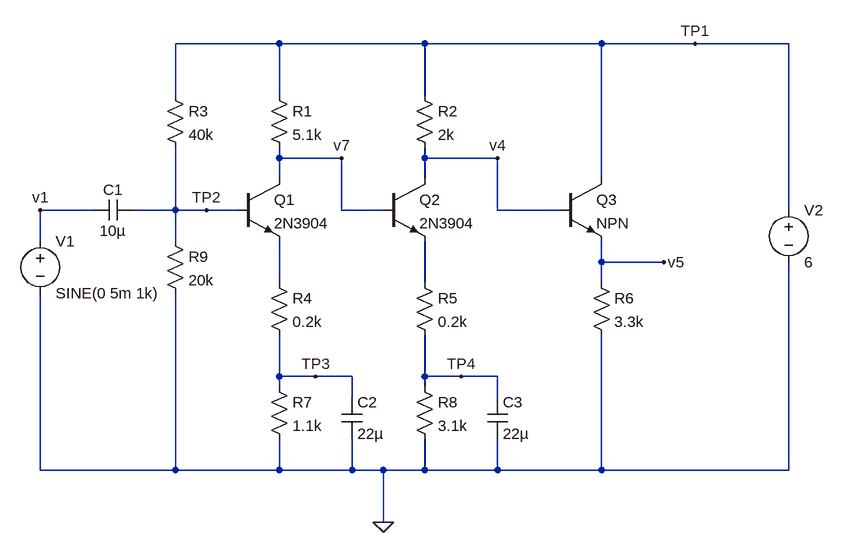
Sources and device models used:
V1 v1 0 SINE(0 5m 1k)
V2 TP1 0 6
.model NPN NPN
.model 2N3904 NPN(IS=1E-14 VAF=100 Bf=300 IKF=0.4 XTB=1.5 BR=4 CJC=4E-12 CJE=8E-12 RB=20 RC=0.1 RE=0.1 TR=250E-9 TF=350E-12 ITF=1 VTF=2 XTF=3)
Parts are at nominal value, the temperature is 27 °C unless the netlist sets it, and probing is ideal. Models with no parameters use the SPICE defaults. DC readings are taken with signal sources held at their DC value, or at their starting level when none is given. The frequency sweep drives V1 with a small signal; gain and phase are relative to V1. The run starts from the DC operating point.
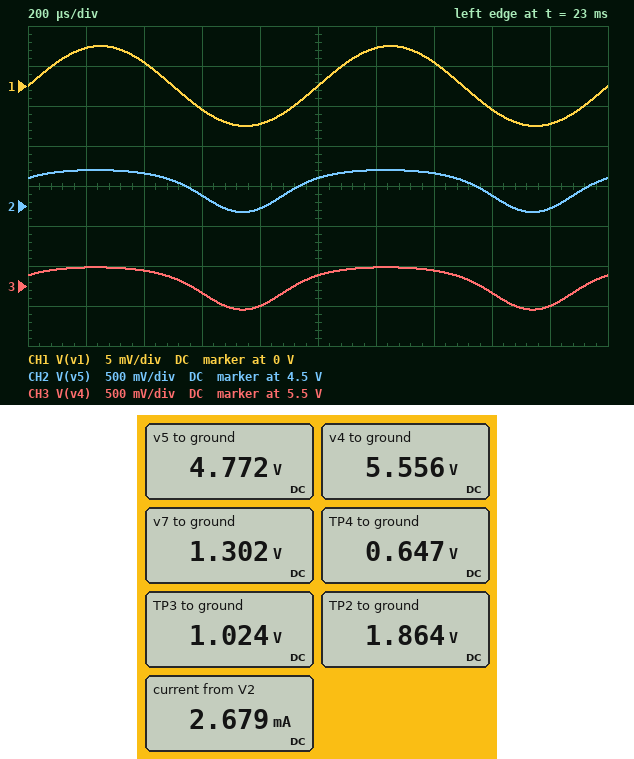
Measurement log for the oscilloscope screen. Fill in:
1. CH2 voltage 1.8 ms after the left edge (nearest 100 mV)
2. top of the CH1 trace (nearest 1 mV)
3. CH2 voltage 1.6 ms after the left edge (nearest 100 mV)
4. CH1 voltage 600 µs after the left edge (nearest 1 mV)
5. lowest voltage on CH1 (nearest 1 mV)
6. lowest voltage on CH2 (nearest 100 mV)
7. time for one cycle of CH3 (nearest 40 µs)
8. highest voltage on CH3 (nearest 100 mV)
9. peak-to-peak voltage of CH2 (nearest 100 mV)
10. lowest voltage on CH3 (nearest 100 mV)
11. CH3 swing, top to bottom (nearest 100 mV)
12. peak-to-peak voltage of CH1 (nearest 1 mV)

4.5 V
5 mV
4.6 V
-3 mV
-5 mV
4.4 V
1.00 ms
5.7 V
500 mV
5.2 V
500 mV
10 mV
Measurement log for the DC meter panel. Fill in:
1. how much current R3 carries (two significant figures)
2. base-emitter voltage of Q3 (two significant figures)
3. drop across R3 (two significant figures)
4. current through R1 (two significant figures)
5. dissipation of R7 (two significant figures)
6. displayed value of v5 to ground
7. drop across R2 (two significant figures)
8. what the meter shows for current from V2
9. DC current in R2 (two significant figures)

100 µA
780 mV
4.1 V
920 µA
950 µW
4.772 V
440 mV
2.679 mA
220 µA
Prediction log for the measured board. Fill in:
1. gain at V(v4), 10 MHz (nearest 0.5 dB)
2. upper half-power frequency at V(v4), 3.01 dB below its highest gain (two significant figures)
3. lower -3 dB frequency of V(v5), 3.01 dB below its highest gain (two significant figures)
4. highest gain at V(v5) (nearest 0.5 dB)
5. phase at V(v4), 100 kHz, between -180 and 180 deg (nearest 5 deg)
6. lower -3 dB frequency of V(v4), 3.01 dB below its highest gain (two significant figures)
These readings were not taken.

14.5 dB
320 kHz
67 Hz
31.5 dB
-20 deg
67 Hz
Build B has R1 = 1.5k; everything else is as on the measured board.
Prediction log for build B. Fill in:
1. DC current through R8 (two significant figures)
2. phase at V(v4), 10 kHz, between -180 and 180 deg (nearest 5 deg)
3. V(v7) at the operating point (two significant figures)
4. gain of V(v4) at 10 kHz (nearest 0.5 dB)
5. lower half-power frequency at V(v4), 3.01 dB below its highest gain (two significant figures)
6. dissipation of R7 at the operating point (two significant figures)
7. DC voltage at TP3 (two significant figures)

1.1 mA
-5 deg
4.4 V
-2.5 dB
17 Hz
1.1 mW
1.1 V
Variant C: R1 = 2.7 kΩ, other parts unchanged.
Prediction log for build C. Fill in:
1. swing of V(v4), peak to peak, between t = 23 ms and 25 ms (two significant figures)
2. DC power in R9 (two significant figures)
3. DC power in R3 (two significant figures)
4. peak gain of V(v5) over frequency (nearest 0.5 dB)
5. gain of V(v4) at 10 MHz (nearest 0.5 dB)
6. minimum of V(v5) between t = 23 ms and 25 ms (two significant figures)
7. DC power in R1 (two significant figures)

970 mV
190 µW
410 µW
39.5 dB
24.0 dB
3.1 V
2.7 mW
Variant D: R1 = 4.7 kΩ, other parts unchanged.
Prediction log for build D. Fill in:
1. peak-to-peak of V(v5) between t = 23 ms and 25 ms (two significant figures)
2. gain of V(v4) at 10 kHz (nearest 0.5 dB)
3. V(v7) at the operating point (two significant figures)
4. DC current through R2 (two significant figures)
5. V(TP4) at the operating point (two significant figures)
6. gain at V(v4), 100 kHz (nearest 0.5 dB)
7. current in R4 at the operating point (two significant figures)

870 mV
38.5 dB
1.4 V
250 µA
740 mV
38.0 dB
980 µA
